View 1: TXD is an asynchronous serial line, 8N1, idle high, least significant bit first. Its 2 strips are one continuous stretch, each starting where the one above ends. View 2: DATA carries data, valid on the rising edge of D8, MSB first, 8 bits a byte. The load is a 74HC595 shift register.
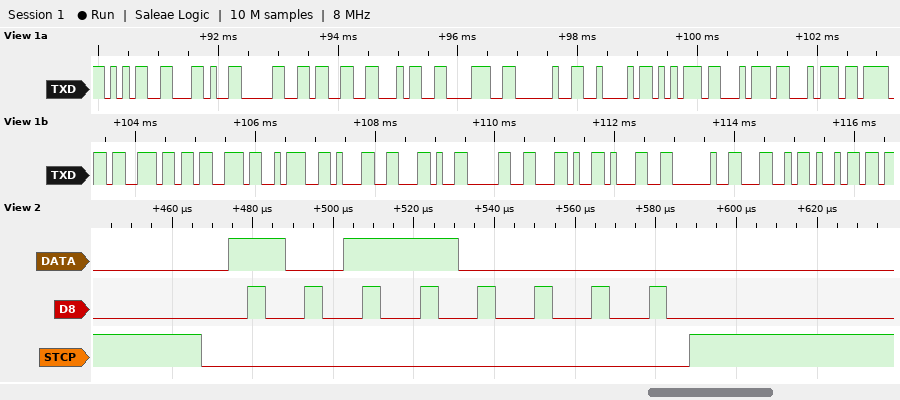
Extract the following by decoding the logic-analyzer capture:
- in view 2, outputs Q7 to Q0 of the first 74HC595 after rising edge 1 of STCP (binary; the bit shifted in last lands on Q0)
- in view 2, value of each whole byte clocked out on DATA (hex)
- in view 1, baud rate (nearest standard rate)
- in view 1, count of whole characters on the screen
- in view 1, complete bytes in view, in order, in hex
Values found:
10110000
0xB0
9600 baud
23
35 2C 30 33 34 38 20 42 75 74 74 6F 6E 73 3A 31 2C 30 2C 31 20 4C 69
